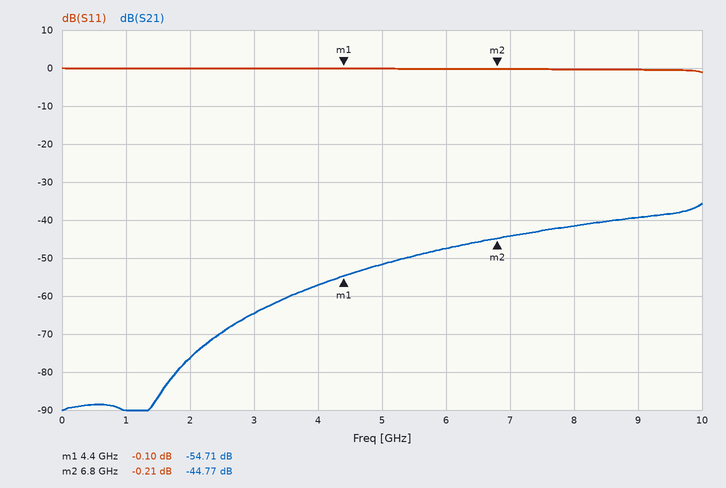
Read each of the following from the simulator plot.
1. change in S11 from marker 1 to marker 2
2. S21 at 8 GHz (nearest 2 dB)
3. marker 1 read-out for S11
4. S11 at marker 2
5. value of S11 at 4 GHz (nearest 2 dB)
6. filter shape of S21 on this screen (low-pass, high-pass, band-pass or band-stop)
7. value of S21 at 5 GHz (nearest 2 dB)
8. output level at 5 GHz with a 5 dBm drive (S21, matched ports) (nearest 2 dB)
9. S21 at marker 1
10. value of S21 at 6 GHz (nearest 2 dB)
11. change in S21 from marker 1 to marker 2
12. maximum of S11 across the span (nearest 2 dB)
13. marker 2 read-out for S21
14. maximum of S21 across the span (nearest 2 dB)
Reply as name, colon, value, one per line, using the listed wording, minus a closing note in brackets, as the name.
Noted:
change in S11 from marker 1 to marker 2: -0.11 dB
S21 at 8 GHz: -42 dB
marker 1 read-out for S11: -0.10 dB
S11 at marker 2: -0.21 dB
value of S11 at 4 GHz: 0 dB
filter shape of S21 on this screen: high-pass
value of S21 at 5 GHz: -52 dB
output level at 5 GHz with a 5 dBm drive (S21, matched ports): -46 dBm
S21 at marker 1: -54.71 dB
value of S21 at 6 GHz: -48 dB
change in S21 from marker 1 to marker 2: 9.94 dB
maximum of S11 across the span: 0 dB
marker 2 read-out for S21: -44.77 dB
maximum of S21 across the span: -36 dB
